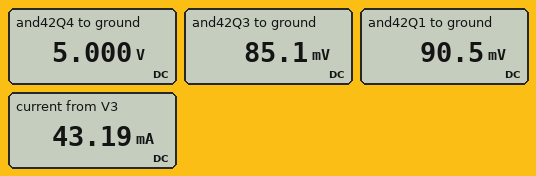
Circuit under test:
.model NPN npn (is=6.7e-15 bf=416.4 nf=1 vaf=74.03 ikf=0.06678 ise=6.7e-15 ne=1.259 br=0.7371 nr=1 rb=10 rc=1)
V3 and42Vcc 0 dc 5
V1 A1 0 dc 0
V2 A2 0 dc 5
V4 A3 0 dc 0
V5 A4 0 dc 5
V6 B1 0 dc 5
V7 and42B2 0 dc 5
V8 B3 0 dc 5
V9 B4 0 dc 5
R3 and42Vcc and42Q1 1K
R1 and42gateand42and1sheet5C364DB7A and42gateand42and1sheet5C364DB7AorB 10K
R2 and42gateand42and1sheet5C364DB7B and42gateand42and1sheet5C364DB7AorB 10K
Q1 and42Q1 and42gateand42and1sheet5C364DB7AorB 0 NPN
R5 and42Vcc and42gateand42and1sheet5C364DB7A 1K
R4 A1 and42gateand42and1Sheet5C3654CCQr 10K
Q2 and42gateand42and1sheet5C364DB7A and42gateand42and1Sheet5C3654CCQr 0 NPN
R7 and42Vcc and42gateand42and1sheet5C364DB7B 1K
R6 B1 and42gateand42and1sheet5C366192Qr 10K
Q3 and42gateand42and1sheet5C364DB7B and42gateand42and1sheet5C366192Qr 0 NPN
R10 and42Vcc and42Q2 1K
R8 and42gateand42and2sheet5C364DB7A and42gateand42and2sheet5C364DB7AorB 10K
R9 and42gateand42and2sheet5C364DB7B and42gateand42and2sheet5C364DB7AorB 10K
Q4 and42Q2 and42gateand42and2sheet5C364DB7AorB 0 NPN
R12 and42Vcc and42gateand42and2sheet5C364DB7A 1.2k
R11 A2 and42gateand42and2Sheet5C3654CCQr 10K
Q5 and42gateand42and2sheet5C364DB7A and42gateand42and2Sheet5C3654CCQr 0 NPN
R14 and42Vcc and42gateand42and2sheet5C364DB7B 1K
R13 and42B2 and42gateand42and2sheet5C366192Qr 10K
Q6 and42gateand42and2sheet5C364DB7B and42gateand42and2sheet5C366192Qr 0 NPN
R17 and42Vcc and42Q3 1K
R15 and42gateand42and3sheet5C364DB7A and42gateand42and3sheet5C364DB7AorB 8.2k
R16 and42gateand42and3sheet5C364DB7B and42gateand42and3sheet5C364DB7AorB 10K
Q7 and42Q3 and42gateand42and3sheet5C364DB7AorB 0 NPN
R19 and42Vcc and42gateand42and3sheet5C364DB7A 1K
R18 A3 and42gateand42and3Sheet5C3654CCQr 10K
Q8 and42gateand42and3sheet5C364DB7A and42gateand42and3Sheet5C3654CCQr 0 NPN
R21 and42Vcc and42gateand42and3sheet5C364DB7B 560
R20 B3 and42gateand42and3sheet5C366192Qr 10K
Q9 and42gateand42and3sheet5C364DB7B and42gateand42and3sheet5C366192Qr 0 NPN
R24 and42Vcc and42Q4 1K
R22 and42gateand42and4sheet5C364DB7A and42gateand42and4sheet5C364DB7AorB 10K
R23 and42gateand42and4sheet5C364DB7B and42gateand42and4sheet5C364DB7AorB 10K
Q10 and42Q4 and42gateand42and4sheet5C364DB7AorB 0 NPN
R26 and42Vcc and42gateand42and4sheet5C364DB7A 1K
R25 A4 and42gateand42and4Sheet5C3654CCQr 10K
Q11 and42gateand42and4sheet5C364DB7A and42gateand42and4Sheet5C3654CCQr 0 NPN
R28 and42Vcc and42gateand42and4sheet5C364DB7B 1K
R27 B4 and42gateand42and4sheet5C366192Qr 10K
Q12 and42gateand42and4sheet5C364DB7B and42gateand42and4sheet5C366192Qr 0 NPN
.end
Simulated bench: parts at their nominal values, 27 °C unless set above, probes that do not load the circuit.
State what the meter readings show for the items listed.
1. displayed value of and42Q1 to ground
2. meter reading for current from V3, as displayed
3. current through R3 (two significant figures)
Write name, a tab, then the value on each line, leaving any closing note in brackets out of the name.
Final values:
displayed value of and42Q1 to ground	90.5 mV
meter reading for current from V3, as displayed	43.19 mA
current through R3	4.9 mA
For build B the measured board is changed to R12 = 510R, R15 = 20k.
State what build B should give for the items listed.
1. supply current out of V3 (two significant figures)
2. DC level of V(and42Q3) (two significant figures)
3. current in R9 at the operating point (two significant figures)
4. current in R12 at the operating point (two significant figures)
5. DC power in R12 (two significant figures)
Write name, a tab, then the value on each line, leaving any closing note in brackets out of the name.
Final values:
supply current out of V3	48 mA
DC level of V(and42Q3)	110 mV
current in R9 at the operating point	1.2 µA
current in R12 at the operating point	9.6 mA
DC power in R12	47 mW
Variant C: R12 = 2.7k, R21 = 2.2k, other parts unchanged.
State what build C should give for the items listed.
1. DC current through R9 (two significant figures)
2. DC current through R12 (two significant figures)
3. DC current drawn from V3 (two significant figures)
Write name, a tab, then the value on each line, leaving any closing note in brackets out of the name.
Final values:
DC current through R9	1.3 µA
DC current through R12	1.8 mA
DC current drawn from V3	34 mA
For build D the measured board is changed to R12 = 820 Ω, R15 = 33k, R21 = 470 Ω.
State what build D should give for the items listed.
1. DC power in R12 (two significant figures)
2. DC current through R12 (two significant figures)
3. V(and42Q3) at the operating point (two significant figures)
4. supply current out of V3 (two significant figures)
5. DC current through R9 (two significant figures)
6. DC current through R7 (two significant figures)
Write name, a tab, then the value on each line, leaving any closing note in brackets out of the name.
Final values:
DC power in R12	29 mW
DC current through R12	6.0 mA
V(and42Q3) at the operating point	140 mV
supply current out of V3	46 mA
DC current through R9	320 nA
DC current through R7	4.9 mA
